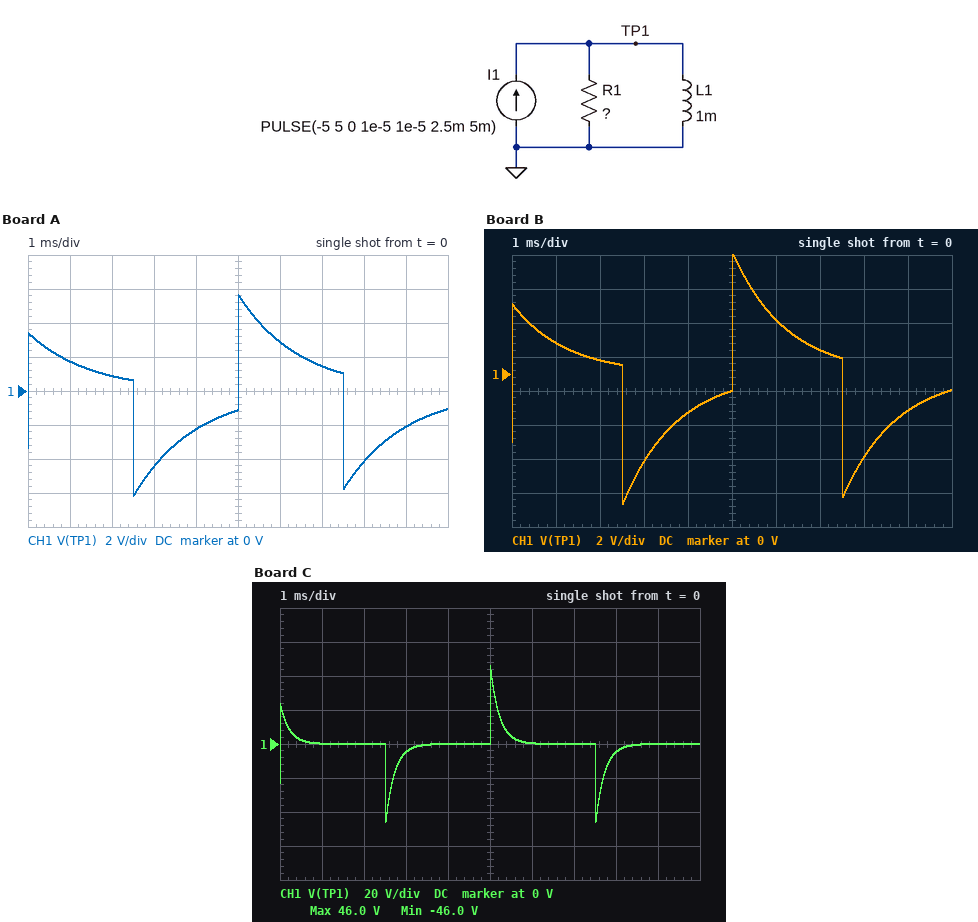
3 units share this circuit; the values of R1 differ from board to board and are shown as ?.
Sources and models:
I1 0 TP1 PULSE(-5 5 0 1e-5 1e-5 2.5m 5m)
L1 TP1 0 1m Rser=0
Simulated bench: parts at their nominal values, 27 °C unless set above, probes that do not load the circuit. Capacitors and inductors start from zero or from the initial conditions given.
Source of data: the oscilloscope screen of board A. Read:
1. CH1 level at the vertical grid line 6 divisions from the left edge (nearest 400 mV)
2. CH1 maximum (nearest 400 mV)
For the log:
2.8 V
5.6 V
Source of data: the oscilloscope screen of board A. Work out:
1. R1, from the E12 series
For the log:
0.68 Ω
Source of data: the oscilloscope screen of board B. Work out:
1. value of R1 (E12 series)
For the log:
0.82 Ω
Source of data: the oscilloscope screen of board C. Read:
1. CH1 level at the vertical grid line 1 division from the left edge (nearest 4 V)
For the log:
0 V
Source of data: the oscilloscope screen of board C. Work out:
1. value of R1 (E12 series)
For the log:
4.7 Ω
